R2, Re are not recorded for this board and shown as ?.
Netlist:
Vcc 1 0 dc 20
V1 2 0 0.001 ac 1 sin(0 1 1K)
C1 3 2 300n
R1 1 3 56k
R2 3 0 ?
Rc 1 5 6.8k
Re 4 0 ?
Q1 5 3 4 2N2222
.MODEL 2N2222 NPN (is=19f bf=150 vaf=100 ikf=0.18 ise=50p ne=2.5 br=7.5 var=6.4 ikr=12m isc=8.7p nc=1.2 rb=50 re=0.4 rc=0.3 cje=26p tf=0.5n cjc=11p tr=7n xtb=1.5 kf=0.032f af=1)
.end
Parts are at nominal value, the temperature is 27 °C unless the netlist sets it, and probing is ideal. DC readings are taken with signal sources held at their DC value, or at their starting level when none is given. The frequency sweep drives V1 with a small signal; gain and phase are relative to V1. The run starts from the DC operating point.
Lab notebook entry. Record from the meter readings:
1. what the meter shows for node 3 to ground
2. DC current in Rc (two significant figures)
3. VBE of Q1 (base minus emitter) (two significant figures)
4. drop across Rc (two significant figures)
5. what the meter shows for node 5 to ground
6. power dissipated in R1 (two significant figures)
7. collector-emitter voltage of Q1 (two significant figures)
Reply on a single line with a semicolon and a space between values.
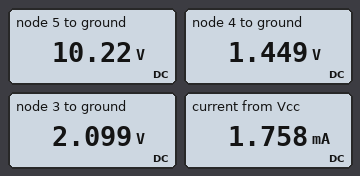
2.099 V; 1.4 mA; 650 mV; 9.8 V; 10.22 V; 5.7 mW; 8.8 V
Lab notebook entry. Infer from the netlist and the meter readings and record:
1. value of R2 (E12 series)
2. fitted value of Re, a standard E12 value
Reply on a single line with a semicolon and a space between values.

6.8 kΩ; 1 kΩ
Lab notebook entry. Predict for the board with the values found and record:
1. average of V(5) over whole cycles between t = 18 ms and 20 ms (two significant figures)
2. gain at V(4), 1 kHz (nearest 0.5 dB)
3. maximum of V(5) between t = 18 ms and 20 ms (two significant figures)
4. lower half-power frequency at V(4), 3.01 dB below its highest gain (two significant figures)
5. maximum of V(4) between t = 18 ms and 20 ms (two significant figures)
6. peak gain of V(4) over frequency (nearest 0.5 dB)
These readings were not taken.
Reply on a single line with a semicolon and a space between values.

10 V; 0 dB; 17 V; 92 Hz; 2.4 V; 0 dB
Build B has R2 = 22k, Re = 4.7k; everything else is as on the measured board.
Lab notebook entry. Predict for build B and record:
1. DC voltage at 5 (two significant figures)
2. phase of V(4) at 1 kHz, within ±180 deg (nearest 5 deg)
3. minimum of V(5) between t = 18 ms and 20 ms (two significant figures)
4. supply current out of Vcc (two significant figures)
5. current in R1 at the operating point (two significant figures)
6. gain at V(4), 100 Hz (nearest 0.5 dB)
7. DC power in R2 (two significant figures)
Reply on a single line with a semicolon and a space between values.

13 V; 0 deg; 12 V; 1.3 mA; 260 µA; -0.5 dB; 1.4 mW
